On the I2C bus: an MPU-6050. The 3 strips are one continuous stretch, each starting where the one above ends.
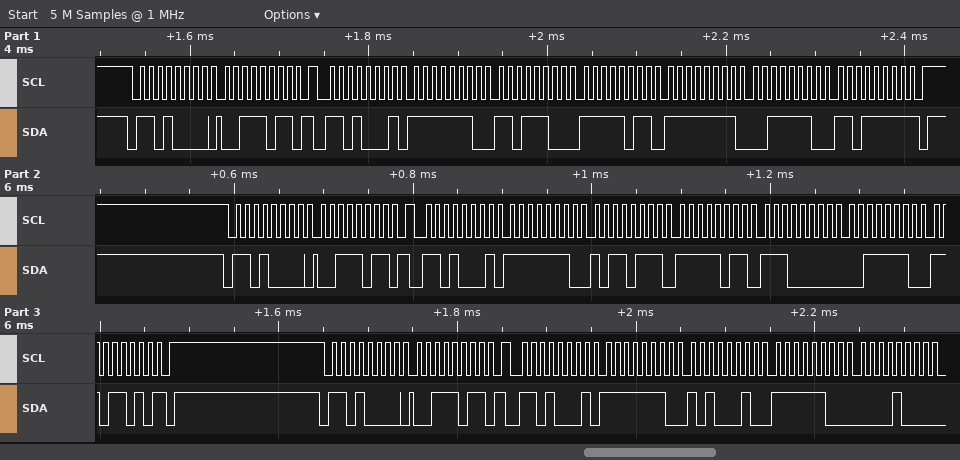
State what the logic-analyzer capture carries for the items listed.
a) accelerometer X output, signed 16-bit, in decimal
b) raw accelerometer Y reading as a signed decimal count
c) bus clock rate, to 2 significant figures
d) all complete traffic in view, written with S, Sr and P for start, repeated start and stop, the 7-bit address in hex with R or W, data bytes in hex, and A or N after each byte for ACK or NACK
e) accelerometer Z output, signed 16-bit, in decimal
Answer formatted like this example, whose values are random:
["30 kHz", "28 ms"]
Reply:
["-292", "-1025", "100 kHz", "S 68W A 3B A Sr 68R A FE A DC A FB A FF A 3E A DF N P S 68W A 3B A Sr 68R A FE A B7 A FB A E0 A 3E A DA N P S 68W A 3B A Sr 68R A FE A A2 A FC A 08 A", "16095"]
